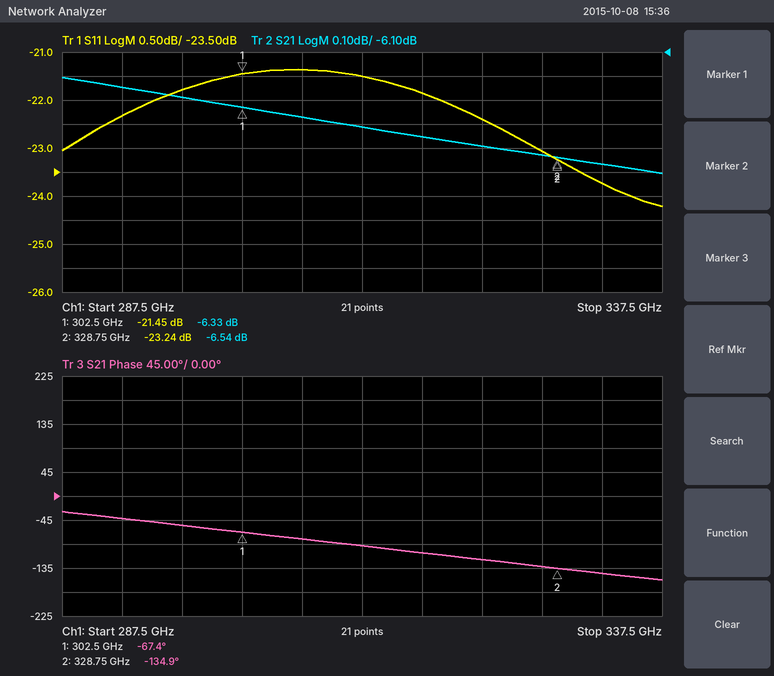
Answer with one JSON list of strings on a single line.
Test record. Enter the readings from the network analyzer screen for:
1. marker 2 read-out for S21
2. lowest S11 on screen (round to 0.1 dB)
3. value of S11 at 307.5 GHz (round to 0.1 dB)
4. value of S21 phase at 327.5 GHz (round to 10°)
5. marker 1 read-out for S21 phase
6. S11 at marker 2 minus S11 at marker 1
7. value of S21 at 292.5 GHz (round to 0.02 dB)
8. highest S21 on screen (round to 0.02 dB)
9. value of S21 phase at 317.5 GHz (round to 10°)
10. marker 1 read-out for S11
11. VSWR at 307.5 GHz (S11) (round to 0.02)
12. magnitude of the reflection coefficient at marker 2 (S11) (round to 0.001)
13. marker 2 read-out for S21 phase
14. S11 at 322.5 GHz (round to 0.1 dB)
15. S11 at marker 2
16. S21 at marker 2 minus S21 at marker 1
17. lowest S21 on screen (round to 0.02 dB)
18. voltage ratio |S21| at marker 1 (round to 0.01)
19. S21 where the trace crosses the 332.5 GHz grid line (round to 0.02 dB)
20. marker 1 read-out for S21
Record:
["-6.54 dB", "-24.2 dB", "-21.4 dB", "-130°", "-67.4°", "-1.79 dB", "-6.24 dB", "-6.20 dB", "-110°", "-21.45 dB", "1.18", "0.069", "-134.9°", "-22.4 dB", "-23.24 dB", "-0.21 dB", "-6.60 dB", "0.48", "-6.56 dB", "-6.33 dB"]
